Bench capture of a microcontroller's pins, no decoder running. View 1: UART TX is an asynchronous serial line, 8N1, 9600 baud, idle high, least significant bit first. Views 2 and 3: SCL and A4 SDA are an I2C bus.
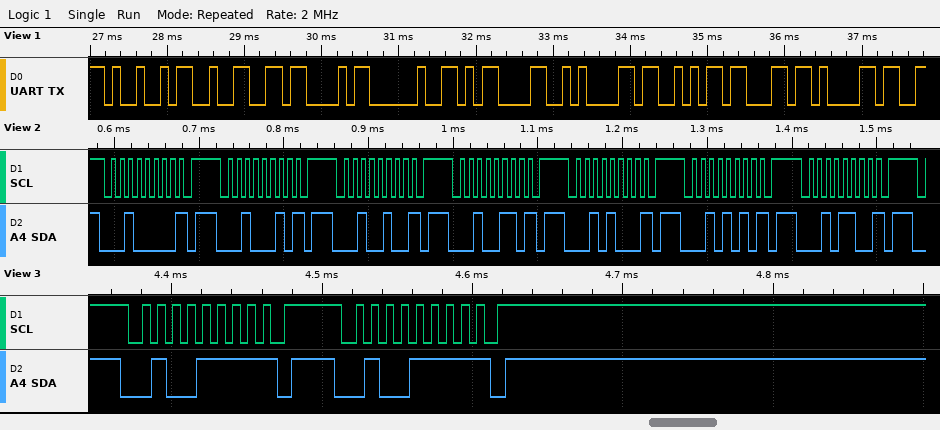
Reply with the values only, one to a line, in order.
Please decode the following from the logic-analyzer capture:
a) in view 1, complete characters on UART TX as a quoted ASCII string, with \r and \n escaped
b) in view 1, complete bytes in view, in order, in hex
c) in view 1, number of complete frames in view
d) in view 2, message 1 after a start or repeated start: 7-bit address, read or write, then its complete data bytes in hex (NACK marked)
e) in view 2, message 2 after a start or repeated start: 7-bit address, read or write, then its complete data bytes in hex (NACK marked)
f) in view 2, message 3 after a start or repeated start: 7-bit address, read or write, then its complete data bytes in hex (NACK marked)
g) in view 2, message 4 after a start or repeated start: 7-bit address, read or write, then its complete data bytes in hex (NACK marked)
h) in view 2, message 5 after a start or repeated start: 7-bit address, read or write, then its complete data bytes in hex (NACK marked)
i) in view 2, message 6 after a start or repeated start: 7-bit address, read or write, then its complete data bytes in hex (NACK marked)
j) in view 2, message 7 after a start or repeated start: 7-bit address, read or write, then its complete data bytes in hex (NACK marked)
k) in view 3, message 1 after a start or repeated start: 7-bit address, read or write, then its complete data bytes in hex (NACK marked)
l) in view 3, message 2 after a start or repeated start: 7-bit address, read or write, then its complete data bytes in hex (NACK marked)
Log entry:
"I2C \r\nSca"
49 32 43 20 0D 0A 53 63 61
9
0x10 write NACK
0x11 write NACK
0x12 write NACK
0x13 write NACK
0x14 write NACK
0x15 write NACK
0x16 write NACK
0x27 read NACK
0x27 read NACK
